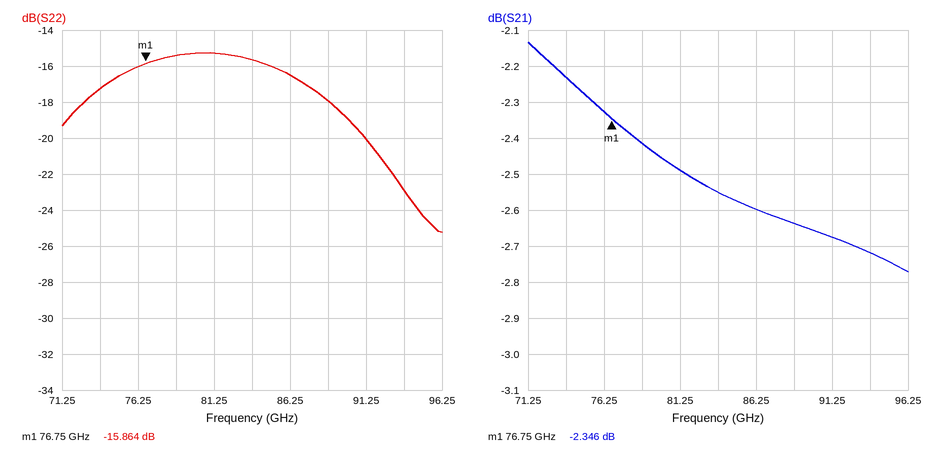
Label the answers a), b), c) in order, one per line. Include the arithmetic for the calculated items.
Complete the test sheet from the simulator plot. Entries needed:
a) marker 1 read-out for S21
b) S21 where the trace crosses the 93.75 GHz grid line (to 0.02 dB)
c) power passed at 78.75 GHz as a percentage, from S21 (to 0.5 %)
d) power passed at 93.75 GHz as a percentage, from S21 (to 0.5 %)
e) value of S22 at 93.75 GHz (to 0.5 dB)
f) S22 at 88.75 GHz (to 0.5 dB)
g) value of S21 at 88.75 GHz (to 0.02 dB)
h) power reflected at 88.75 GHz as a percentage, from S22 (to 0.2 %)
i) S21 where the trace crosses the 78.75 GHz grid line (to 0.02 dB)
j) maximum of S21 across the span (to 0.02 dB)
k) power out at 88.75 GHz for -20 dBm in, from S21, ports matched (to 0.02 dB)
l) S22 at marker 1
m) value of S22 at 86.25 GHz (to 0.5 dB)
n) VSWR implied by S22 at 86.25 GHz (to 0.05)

a) -2.346 dB
b) -2.72 dB
c) 10^(-2.42/10) ≈ 57.3 %, so 57.5 % to the nearest 0.5 %
d) 10^(-2.72/10) ≈ 53.5 %
e) -23.0 dB
f) -18.0 dB
g) -2.64 dB
h) 10^(-18/10) ≈ 1.6 %
i) -2.42 dB
j) -2.14 dB
k) -20 dBm + (-2.64 dB) = -22.64 dBm
l) -15.864 dB
m) -16.5 dB
n) |Γ| = 10^(-16.5/20) = 0.1496; VSWR = (1 + 0.1496)/(1 − 0.1496) ≈ 1.35
